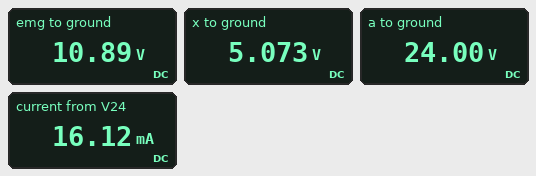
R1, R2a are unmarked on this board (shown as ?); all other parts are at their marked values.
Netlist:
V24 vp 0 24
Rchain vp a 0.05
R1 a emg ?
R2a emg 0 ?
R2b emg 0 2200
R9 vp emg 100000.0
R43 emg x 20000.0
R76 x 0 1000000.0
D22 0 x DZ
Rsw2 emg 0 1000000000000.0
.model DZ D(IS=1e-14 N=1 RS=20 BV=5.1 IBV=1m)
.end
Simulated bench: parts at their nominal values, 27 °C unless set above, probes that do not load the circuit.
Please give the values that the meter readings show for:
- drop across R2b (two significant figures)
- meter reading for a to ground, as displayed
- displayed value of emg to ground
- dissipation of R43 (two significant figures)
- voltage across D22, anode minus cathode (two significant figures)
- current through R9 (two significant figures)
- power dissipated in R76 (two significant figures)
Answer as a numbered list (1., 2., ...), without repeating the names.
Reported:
1. 11 V
2. 24.00 V
3. 10.89 V
4. 1.7 mW
5. -5.1 V
6. 130 µA
7. 26 µW
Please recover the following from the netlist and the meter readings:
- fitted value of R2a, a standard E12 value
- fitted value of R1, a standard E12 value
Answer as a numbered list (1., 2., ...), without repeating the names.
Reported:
1. 1 kΩ
2. 820 Ω
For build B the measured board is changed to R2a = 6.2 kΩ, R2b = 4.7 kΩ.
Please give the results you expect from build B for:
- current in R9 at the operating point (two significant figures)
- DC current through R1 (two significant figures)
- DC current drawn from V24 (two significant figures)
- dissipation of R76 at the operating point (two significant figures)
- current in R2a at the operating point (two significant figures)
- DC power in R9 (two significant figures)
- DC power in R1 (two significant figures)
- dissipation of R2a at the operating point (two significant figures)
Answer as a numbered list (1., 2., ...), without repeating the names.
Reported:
1. 60 µA
2. 7.3 mA
3. 7.4 mA
4. 26 µW
5. 2.9 mA
6. 360 µW
7. 44 mW
8. 52 mW
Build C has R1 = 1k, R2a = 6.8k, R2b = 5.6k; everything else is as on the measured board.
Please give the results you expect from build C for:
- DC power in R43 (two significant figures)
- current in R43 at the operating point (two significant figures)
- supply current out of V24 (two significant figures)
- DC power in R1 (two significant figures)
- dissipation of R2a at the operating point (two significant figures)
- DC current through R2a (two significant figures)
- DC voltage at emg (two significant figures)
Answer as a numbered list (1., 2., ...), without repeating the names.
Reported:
1. 7.9 mW
2. 630 µA
3. 6.4 mA
4. 40 mW
5. 46 mW
6. 2.6 mA
7. 18 V
